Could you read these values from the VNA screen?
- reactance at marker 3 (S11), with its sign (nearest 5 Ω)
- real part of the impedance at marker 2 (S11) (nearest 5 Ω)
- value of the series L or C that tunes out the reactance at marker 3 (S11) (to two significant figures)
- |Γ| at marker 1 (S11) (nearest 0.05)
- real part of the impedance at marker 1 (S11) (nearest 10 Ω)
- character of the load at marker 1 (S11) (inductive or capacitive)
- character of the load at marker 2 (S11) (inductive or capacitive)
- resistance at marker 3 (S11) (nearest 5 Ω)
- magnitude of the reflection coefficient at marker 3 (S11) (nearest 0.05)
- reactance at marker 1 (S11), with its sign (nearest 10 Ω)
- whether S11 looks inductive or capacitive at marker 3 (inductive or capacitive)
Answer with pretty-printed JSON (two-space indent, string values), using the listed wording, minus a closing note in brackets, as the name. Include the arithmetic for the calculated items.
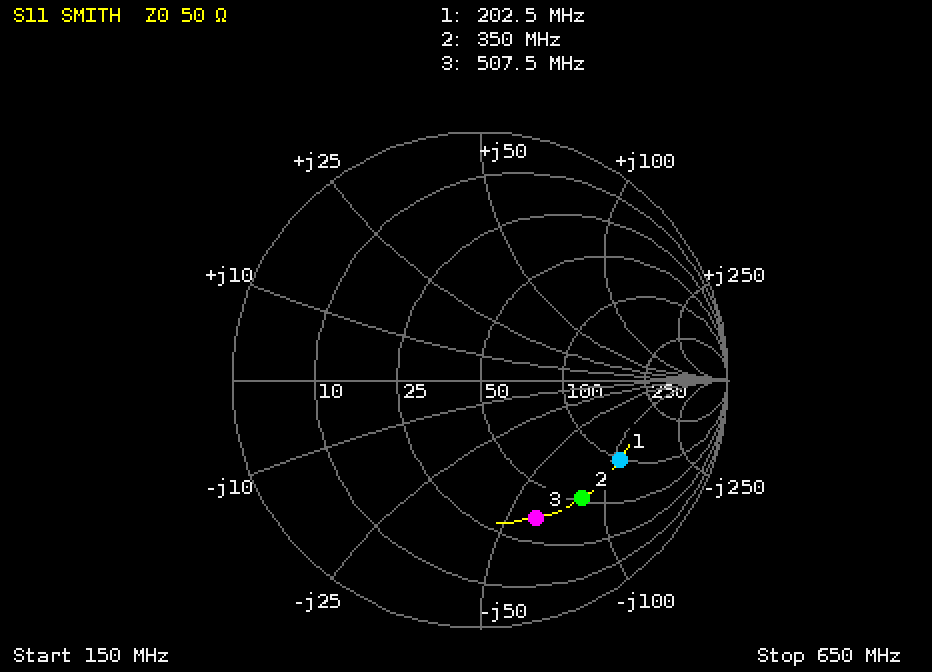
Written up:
{
  "reactance at marker 3 (S11), with its sign": "-60 Ω",
  "real part of the impedance at marker 2 (S11)": "55 Ω",
  "value of the series L or C that tunes out the reactance at marker 3 (S11)": "L = 60 Ω/(2π × 507.5 MHz) ≈ 19 nH",
  "|Γ| at marker 1 (S11)": "0.65",
  "real part of the impedance at marker 1 (S11)": "100 Ω",
  "character of the load at marker 1 (S11)": "capacitive",
  "character of the load at marker 2 (S11)": "capacitive",
  "resistance at marker 3 (S11)": "35 Ω",
  "magnitude of the reflection coefficient at marker 3 (S11)": "0.60",
  "reactance at marker 1 (S11), with its sign": "-110 Ω",
  "whether S11 looks inductive or capacitive at marker 3": "capacitive"
}
